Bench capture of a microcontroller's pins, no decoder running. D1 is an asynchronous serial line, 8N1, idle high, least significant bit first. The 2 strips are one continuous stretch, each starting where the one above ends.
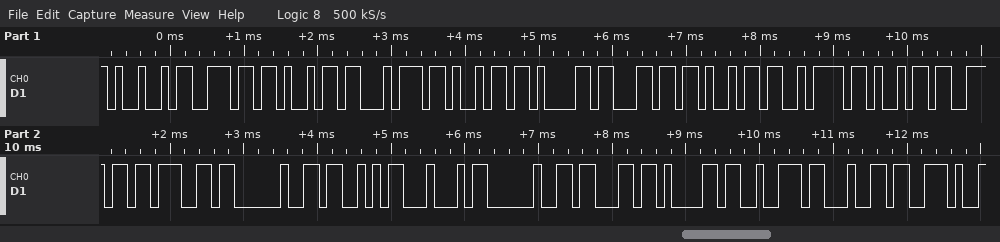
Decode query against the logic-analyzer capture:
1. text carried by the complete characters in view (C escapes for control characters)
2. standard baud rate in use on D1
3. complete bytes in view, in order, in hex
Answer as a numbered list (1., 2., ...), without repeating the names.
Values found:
1. "Initializing SD card."
2. 9600 baud
3. 0x49 0x6E 0x69 0x74 0x69 0x61 0x6C 0x69 0x7A 0x69 0x6E 0x67 0x20 0x53 0x44 0x20 0x63 0x61 0x72 0x64 0x2E
